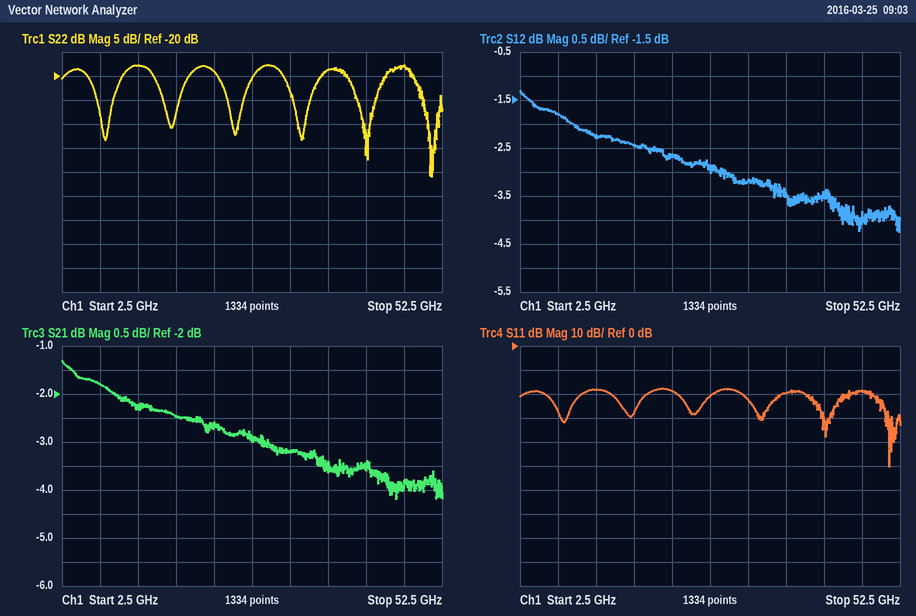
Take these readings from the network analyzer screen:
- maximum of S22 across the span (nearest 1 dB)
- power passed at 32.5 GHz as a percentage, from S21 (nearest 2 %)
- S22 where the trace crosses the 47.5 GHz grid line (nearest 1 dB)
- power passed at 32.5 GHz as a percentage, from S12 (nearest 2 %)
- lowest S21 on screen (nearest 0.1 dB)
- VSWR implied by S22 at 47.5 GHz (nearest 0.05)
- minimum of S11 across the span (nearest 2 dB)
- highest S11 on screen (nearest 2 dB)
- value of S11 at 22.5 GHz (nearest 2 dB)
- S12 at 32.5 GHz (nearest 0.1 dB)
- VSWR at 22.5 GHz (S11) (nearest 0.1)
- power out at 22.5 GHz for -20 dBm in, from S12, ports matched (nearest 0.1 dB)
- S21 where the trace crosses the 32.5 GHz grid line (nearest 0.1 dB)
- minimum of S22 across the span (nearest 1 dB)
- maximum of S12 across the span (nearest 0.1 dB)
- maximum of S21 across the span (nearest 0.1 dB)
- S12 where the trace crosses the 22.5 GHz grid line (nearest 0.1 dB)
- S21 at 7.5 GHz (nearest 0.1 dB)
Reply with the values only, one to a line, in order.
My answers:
-18 dB
48 %
-18 dB
48 %
-4.2 dB
1.30
-50 dB
-18 dB
-18 dB
-3.2 dB
1.3
-22.7 dBm
-3.2 dB
-41 dB
-1.3 dB
-1.3 dB
-2.7 dB
-1.8 dB
